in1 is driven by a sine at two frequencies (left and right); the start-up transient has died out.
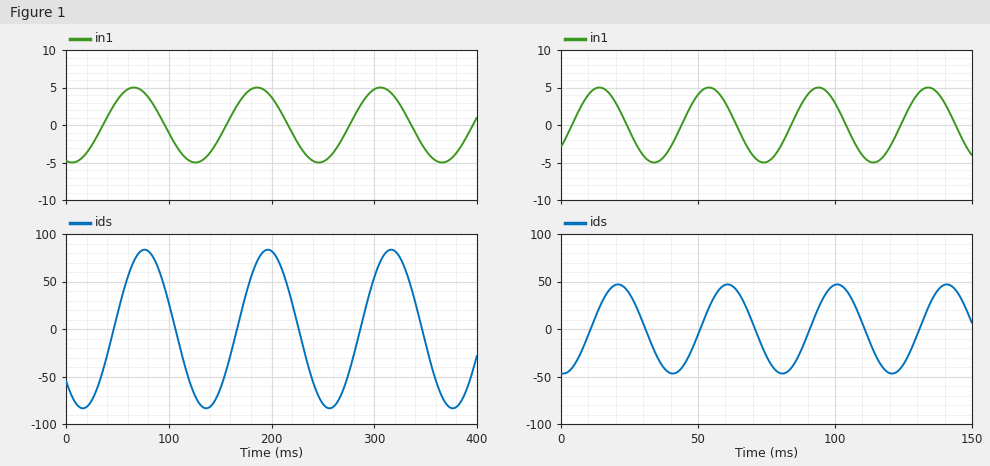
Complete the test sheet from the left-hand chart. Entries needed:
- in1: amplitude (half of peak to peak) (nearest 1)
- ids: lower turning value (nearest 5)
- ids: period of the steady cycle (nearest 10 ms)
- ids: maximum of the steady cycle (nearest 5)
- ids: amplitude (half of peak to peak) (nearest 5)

5
-85
120 ms
85
85
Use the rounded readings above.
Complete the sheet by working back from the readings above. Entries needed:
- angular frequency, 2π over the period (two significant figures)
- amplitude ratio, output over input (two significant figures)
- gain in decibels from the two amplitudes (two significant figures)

0.052 rad/ms
17
25 dB
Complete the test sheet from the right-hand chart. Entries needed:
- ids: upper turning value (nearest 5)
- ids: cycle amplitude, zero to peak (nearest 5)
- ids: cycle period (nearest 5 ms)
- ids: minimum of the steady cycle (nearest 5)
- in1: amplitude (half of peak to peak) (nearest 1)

45
45
40 ms
-45
5
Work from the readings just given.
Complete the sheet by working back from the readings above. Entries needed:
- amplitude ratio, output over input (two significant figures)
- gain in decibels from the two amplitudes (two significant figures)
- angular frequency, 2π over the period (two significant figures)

9.0
19 dB
0.16 rad/ms
